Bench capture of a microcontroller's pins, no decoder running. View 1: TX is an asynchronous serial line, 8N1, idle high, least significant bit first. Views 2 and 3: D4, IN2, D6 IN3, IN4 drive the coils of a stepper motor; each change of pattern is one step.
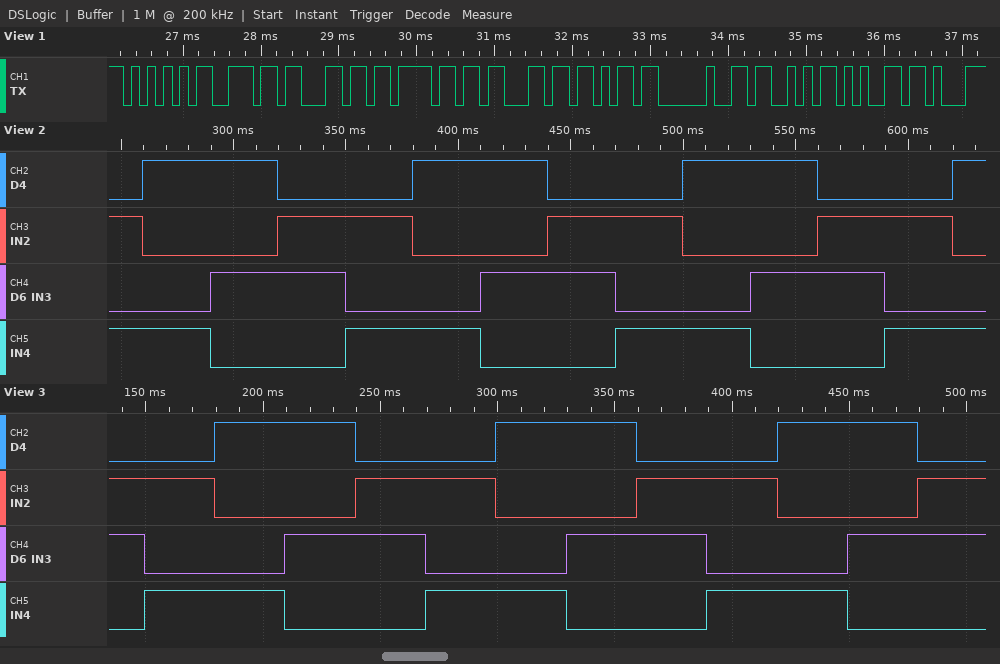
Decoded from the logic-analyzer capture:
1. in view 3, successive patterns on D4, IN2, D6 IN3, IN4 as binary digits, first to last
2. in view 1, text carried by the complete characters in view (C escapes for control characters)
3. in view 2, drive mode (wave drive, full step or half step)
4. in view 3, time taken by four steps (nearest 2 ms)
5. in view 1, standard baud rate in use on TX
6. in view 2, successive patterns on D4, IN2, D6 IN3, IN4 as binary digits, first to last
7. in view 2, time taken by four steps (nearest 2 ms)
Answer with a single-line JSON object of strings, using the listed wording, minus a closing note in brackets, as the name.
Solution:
{"in view 3, successive patterns on D4, IN2, D6 IN3, IN4 as binary digits, first to last": "0110 0101 1001 1010 0110 0101 1001 1010 0110 0101 1001 1010 0110", "in view 1, text carried by the complete characters in view": "\"Unlock Se\"", "in view 2, drive mode": "full step", "in view 3, time taken by four steps": "120 ms", "in view 1, standard baud rate in use on TX": "9600 baud", "in view 2, successive patterns on D4, IN2, D6 IN3, IN4 as binary digits, first to last": "0101 1001 1010 0110 0101 1001 1010 0110 0101 1001 1010 0110 0101 1001", "in view 2, time taken by four steps": "120 ms"}
